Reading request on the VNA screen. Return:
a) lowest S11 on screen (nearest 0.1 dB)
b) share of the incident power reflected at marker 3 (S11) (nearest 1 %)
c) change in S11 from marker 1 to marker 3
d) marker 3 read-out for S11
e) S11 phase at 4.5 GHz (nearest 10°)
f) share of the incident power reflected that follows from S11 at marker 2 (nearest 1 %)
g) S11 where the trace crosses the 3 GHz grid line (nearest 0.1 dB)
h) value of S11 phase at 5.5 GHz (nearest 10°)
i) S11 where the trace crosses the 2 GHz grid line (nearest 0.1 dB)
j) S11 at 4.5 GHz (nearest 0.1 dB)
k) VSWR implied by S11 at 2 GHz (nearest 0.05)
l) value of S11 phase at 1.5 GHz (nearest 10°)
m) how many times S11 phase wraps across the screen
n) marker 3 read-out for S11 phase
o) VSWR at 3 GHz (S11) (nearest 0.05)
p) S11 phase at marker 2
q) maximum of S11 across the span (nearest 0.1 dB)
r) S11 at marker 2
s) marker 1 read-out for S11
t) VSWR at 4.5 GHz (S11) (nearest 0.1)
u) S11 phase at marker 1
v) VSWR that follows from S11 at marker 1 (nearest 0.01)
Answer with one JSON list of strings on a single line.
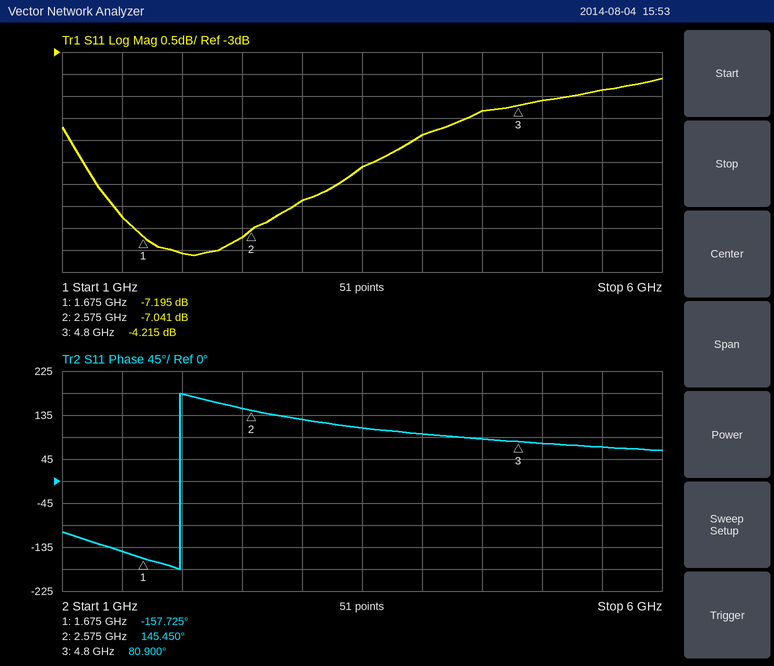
["-7.6 dB", "38 %", "2.980 dB", "-4.215 dB", "90°", "20 %", "-6.4 dB", "70°", "-7.6 dB", "-4.3 dB", "2.45", "-140°", "1", "80.900°", "2.85", "145.450°", "-3.6 dB", "-7.041 dB", "-7.195 dB", "4.1", "-157.725°", "2.55"]
